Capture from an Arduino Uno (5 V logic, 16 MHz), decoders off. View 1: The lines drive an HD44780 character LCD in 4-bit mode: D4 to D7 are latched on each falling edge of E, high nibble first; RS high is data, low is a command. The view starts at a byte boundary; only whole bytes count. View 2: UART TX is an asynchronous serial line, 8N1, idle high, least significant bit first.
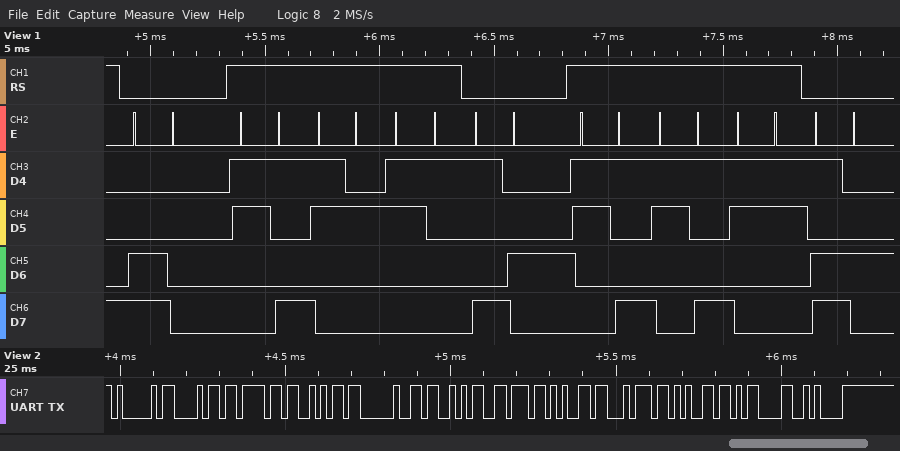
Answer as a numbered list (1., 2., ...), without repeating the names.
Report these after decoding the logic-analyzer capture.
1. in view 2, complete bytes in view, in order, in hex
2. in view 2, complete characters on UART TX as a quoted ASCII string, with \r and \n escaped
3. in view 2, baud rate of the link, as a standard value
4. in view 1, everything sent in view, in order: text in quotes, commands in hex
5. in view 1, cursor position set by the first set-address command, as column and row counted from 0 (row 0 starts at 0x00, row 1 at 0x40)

1. 41 68 6F 6A 20 53 76 65 74 65 0D 0A
2. "Ahoj Svete\r\n"
3. 57600 baud
4. 0xC0 "921" 0x94 "993" 0xD4
5. column 0, row 1
